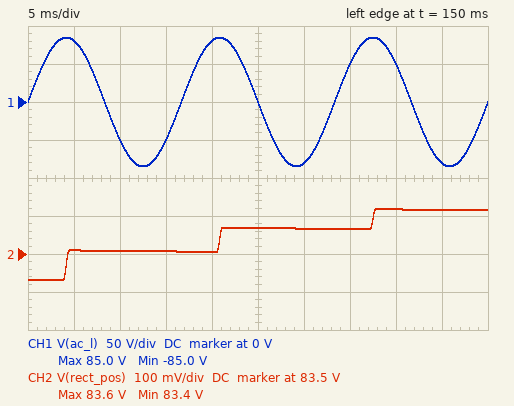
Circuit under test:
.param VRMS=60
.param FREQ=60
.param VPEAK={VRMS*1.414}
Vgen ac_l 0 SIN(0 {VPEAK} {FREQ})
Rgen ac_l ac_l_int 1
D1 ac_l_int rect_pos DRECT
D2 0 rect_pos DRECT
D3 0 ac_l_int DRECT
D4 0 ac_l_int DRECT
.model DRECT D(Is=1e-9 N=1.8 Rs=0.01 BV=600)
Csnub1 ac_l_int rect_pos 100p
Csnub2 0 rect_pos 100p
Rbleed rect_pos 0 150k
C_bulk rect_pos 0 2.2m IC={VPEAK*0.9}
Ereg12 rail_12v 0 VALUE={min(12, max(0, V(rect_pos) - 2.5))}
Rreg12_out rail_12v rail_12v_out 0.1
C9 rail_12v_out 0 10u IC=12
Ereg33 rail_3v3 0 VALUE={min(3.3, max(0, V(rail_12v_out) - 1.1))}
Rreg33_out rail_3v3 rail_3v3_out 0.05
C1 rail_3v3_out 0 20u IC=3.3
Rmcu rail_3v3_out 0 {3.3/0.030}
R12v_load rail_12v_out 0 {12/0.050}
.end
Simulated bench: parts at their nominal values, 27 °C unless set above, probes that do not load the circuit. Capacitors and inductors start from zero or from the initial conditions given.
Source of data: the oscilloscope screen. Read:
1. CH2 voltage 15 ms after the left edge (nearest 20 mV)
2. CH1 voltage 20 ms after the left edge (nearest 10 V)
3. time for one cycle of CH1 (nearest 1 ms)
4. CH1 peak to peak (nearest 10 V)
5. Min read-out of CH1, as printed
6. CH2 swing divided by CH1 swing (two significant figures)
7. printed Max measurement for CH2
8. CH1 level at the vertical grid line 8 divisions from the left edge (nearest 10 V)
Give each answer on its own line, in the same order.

83.50 V
80 V
17 ms
170 V
-85.0 V
0.0011
83.6 V
50 V
